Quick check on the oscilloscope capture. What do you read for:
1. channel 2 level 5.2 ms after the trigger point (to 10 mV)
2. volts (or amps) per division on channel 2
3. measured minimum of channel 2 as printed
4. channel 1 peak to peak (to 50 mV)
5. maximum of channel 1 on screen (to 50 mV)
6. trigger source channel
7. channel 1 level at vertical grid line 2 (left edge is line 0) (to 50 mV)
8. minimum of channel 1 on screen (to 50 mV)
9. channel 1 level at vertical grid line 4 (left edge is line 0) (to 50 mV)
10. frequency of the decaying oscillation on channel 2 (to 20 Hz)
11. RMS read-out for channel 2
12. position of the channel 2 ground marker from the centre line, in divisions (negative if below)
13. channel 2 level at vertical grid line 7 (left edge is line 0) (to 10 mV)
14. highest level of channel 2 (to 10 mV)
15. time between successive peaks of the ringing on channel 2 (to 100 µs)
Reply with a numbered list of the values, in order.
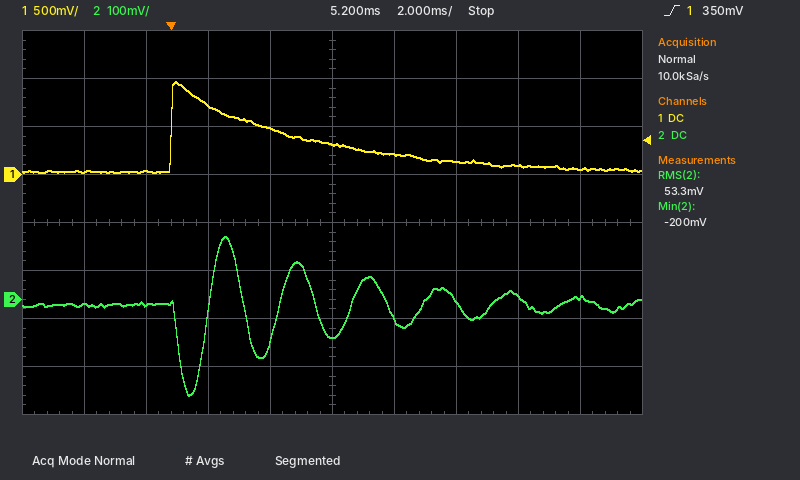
1. -80 mV
2. 100 mV
3. -200 mV
4. 950 mV
5. 950 mV
6. channel 1
7. 50 mV
8. 0 mV
9. 500 mV
10. 440 Hz
11. 53.3 mV
12. -1.6 div
13. 0 mV
14. 130 mV
15. 2.3 ms
